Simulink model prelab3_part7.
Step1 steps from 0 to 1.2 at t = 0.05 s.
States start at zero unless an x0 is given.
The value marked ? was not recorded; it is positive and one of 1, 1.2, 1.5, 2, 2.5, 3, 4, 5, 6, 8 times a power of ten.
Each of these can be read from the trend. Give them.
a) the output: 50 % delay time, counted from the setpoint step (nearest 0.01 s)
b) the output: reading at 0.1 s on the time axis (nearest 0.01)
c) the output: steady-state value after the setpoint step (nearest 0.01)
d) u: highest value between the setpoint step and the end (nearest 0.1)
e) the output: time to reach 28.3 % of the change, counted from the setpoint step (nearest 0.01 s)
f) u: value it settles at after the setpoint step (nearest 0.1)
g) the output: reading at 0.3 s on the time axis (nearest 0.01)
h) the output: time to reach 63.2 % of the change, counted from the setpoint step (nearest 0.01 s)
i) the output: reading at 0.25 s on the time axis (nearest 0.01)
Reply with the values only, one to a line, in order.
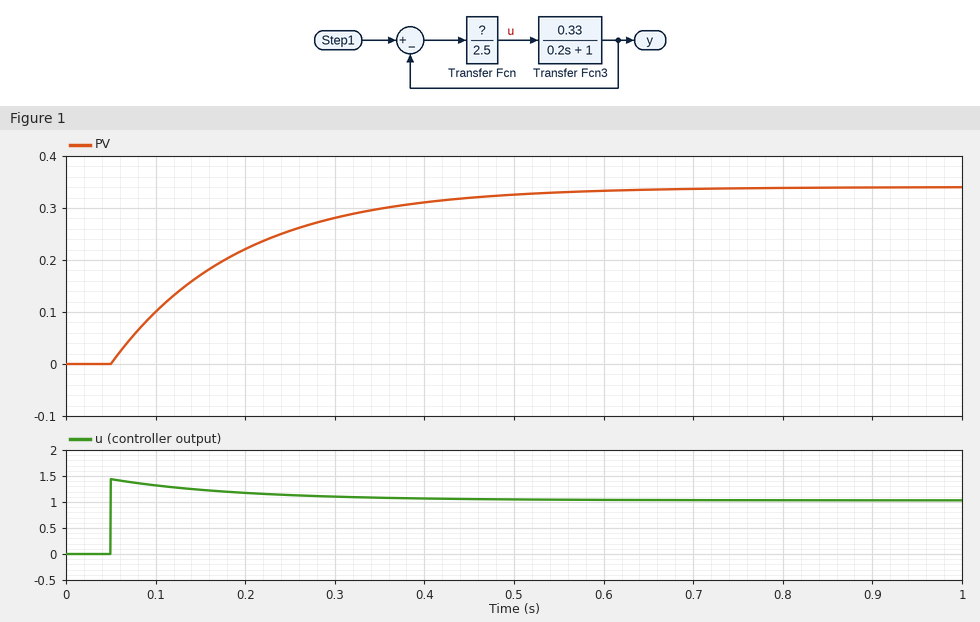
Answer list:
0.10 s
0.10
0.34
1.4
0.05 s
1.0
0.28
0.14 s
0.26
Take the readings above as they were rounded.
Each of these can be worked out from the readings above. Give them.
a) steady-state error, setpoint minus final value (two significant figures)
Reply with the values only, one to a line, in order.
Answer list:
0.86
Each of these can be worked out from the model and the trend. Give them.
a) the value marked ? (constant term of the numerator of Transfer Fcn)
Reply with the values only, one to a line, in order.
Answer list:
3
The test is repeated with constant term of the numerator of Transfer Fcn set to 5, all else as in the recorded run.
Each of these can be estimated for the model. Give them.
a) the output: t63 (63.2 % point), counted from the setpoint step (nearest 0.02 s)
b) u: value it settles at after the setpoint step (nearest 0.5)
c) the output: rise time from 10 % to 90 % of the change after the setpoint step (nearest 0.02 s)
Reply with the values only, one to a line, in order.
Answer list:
0.12 s
1.5
0.26 s
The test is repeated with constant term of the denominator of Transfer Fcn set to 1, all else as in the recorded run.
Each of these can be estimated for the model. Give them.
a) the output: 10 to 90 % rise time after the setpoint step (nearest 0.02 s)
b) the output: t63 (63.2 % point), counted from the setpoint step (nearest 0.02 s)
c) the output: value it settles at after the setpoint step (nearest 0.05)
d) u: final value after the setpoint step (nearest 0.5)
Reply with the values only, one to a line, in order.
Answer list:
0.22 s
0.10 s
0.60
2.0
